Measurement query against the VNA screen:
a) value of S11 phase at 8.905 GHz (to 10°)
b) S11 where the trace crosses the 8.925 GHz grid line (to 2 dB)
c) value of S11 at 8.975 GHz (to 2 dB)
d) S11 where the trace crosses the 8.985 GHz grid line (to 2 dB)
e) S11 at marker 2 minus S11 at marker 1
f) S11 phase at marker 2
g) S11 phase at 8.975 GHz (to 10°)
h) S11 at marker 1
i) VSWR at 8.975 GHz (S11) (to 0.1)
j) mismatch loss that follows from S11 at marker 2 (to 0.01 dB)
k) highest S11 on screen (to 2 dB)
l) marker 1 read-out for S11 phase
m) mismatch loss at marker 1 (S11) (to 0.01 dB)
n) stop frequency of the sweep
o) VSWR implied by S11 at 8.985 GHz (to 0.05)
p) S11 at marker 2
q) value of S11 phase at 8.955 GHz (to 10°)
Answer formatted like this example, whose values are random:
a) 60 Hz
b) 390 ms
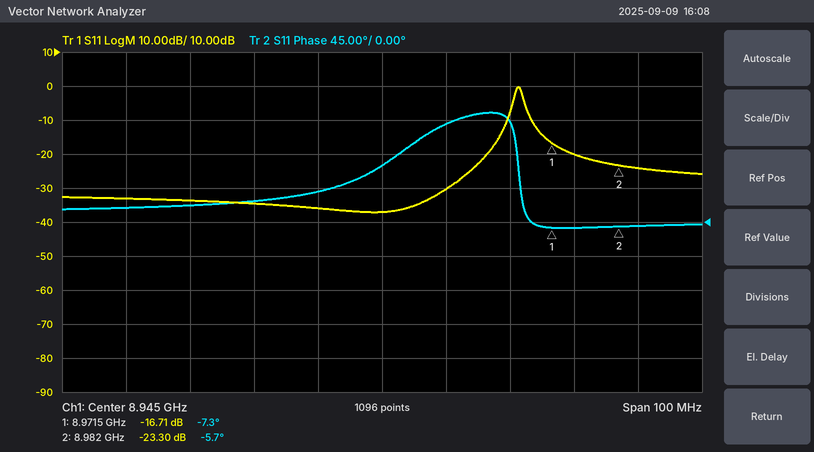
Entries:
a) 20°
b) -34 dB
c) -20 dB
d) -24 dB
e) -6.59 dB
f) -5.7°
g) -10°
h) -16.71 dB
i) 1.2
j) 0.02 dB
k) 0 dB
l) -7.3°
m) 0.09 dB
n) 8.995 GHz
o) 1.15
p) -23.30 dB
q) 130°
